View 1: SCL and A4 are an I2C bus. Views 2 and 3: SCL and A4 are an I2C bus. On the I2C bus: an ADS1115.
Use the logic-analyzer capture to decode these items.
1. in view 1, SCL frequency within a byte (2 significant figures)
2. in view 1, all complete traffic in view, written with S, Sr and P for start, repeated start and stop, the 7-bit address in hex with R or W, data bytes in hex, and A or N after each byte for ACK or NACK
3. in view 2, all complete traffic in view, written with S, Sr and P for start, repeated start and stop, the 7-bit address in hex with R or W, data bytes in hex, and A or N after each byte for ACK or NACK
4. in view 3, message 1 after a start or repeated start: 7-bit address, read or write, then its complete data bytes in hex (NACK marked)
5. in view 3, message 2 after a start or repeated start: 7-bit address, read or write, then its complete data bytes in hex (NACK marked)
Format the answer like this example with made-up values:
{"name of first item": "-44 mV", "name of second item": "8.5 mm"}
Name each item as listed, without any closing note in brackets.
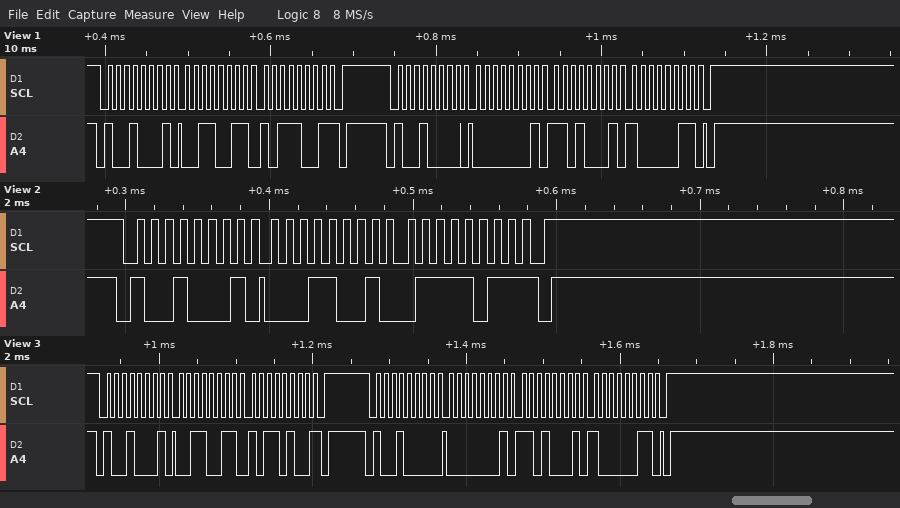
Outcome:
{"in view 1, SCL frequency within a byte": "100 kHz", "in view 1, all complete traffic in view, written with S, Sr and P for start, repeated start and stop, the 7-bit address in hex with R or W, data bytes in hex, and A or N after each byte for ACK or NACK": "S 48R A 33 A B9 N P S 48W A 01 A D1 A 83 A P", "in view 2, all complete traffic in view, written with S, Sr and P for start, repeated start and stop, the 7-bit address in hex with R or W, data bytes in hex, and A or N after each byte for ACK or NACK": "S 48R A 19 A 7B N P", "in view 3, message 1 after a start or repeated start: 7-bit address, read or write, then its complete data bytes in hex": "0x48 read: 33 B4 NACK", "in view 3, message 2 after a start or repeated start: 7-bit address, read or write, then its complete data bytes in hex": "0x48 write: 01 D1 83"}
